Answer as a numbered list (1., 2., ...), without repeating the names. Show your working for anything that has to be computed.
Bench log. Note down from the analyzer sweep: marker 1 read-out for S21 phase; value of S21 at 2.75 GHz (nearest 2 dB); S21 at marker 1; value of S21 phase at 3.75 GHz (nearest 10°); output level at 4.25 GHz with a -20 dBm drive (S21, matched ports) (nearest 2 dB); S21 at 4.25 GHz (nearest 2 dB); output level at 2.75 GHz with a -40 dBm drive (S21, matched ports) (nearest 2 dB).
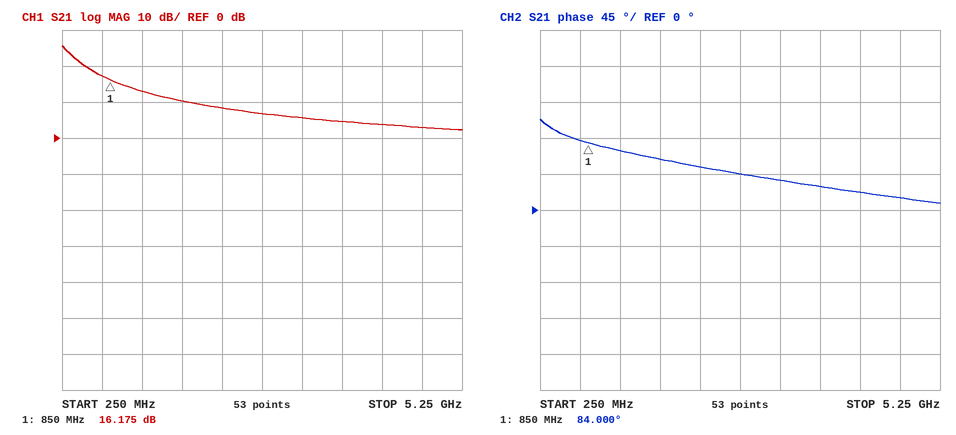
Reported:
1. 84.000°
2. 6 dB
3. 16.175 dB
4. 30°
5. -20 dBm + (4 dB) = -16 dBm
6. 4 dB
7. -40 dBm + (6 dB) = -34 dBm
